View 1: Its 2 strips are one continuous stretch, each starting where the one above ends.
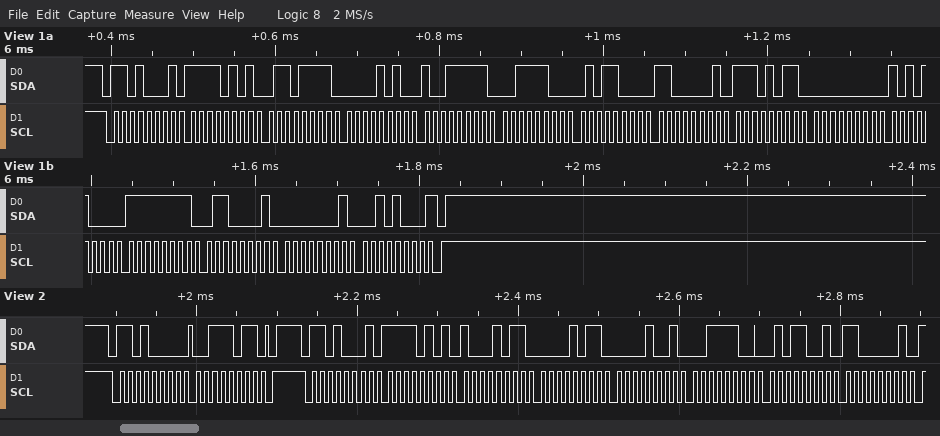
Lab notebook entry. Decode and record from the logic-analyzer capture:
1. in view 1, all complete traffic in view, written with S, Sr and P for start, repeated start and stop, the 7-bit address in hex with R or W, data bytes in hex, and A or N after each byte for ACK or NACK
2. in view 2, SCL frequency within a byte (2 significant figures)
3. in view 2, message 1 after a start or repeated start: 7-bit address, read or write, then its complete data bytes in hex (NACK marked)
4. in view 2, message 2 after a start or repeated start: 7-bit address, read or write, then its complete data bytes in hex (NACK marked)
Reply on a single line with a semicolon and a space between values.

S 68R A F5 A 6F A 0A A 9F A 3C A 58 A C1 A EB A 00 A A8 A FF A 61 A 01 A 28 N P; 100 kHz; 0x68 write: 3B; 0x68 read: F5 8B 0B 09 3C 59 C1
